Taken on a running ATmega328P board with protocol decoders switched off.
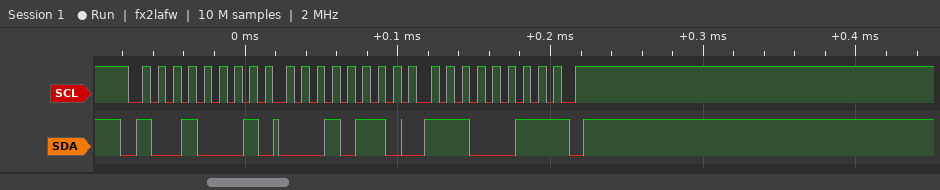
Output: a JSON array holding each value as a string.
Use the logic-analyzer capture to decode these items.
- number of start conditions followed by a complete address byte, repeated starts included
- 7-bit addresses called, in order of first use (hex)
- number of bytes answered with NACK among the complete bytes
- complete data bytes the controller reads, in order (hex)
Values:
["1", "0x48", "1", "16 E3"]
